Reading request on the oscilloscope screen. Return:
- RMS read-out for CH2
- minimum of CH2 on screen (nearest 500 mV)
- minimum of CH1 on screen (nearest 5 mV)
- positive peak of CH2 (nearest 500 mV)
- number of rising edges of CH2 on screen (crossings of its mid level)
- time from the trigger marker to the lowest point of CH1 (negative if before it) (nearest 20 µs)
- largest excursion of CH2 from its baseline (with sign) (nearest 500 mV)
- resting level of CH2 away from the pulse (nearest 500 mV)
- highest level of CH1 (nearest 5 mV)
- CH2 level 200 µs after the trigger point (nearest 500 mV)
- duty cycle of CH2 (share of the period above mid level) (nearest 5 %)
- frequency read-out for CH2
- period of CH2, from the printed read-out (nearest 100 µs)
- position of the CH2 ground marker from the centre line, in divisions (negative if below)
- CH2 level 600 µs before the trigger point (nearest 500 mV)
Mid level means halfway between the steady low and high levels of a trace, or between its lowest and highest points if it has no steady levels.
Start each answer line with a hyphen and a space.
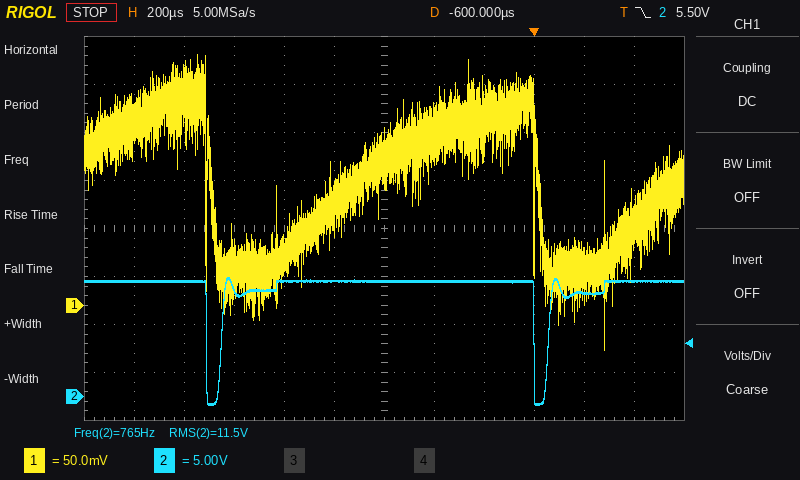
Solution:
- 11.5 V
- -1.0 V
- -45 mV
- 12.5 V
- 2
- +280 µs
- -13.0 V
- 12.0 V
- 260 mV
- 11.0 V
- 95 %
- 765 Hz
- 1.3 ms
- -3.5 div
- 12.0 V
